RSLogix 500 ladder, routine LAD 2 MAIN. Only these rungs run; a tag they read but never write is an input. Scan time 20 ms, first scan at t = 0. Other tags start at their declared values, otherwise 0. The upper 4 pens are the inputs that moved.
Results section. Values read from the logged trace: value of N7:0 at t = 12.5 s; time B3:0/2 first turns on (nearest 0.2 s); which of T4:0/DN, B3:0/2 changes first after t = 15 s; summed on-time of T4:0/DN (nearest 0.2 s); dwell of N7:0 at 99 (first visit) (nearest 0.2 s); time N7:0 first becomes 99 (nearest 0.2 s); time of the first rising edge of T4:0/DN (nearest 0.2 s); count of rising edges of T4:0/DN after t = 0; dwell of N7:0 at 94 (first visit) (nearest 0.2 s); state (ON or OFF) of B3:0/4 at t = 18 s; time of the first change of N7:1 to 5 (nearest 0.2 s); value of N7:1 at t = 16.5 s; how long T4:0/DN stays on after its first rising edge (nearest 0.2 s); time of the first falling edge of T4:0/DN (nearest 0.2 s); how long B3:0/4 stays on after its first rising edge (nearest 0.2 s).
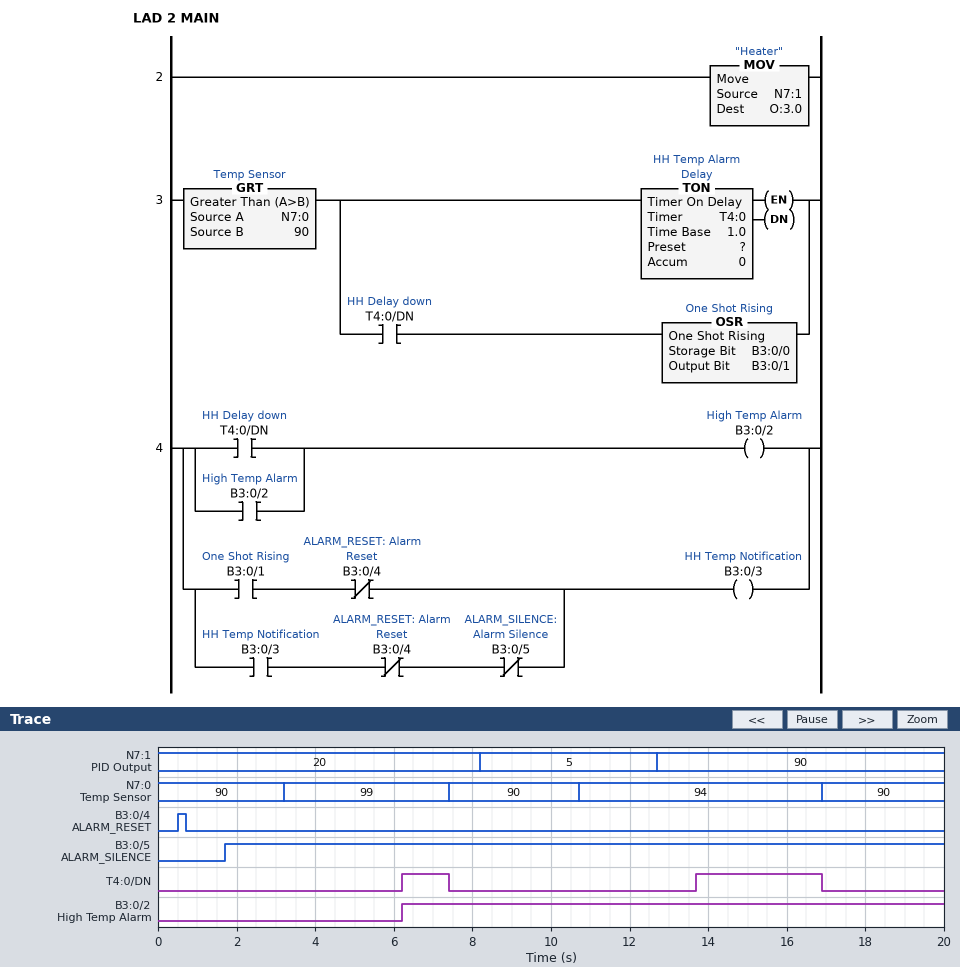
94
6.2 s
T4:0/DN
4.4 s
4.2 s
3.2 s
6.2 s
2
6.2 s
OFF
8.2 s
90
1.2 s
7.4 s
0.2 s
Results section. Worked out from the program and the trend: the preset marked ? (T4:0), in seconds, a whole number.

3 s
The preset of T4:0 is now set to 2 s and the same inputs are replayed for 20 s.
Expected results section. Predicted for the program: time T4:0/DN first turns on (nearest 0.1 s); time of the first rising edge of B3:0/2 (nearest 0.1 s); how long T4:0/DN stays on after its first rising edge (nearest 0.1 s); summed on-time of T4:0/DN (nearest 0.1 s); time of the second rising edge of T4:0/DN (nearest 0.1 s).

5.2 s
5.2 s
2.2 s
6.4 s
12.7 s
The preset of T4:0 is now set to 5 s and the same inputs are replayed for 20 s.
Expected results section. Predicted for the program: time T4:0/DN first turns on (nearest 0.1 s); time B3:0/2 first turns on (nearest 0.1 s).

15.7 s
15.7 s
